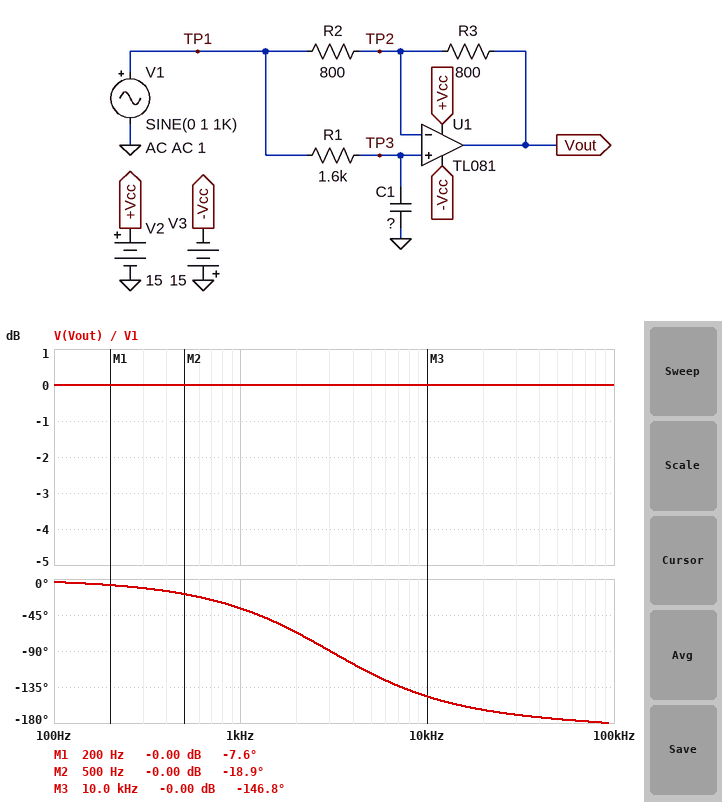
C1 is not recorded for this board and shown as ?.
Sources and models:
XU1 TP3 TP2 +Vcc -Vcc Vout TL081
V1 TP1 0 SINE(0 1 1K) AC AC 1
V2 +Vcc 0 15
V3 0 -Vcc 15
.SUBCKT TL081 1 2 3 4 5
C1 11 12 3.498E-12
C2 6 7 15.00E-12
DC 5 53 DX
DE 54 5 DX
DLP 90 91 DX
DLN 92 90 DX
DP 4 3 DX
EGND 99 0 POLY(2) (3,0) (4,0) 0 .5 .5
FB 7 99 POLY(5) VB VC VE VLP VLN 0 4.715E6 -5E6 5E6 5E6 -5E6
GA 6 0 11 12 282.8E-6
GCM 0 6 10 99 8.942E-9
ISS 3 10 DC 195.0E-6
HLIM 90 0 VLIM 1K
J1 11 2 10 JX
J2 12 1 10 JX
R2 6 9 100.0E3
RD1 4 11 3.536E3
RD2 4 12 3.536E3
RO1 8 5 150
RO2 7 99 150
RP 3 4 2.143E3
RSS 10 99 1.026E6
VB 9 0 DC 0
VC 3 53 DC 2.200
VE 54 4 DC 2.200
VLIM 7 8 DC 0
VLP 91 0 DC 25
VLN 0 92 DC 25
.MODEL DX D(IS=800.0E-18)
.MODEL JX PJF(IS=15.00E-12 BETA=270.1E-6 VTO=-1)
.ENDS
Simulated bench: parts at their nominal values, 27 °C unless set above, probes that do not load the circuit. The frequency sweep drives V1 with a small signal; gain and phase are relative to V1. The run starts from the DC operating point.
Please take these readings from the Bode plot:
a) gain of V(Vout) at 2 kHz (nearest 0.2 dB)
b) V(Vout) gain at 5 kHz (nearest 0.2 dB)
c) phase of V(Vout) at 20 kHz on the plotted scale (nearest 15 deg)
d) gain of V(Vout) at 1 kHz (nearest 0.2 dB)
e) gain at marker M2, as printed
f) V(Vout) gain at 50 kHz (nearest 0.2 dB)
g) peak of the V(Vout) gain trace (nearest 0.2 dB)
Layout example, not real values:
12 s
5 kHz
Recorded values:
0 dB
0 dB
-165 deg
0 dB
-0.00 dB
0 dB
0 dB
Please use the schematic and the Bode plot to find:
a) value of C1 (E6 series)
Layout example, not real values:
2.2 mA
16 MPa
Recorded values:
33 nF
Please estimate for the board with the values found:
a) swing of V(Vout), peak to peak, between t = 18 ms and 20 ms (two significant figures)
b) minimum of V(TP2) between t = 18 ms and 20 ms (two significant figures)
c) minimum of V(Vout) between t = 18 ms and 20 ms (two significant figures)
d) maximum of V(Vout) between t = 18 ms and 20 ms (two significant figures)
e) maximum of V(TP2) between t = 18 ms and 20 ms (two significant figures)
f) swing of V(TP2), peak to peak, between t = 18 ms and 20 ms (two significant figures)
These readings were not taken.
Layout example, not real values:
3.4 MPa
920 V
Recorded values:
2.0 V
-950 mV
-1.0 V
1.0 V
950 mV
1.9 V
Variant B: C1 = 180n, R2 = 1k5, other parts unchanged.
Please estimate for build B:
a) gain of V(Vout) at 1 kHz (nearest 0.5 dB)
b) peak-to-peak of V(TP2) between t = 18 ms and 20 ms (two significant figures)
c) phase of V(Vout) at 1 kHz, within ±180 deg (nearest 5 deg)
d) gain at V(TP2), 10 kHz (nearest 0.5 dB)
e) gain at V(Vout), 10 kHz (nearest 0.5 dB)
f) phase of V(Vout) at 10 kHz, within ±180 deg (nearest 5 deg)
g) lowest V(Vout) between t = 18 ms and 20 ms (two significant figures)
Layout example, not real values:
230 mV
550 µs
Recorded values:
-3.5 dB
970 mV
-105 deg
-25.5 dB
-5.5 dB
-170 deg
-670 mV
